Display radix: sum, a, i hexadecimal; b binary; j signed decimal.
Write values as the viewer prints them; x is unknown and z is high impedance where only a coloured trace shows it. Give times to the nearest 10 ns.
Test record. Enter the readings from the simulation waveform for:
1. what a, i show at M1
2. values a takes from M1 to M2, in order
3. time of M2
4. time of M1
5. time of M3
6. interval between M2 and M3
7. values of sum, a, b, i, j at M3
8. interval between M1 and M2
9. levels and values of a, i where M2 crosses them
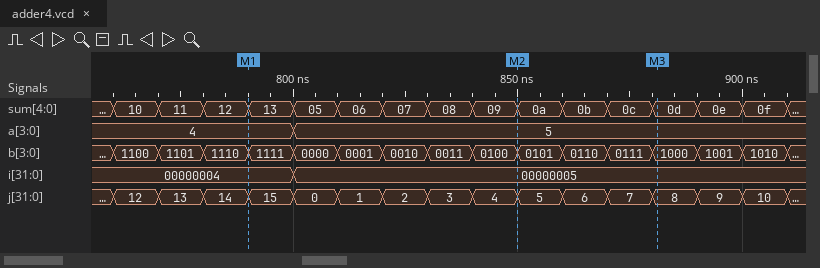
a=4, i=00000004
4, 5
850 ns
790 ns
880 ns
30 ns
sum=0d, a=5, b=1000, i=00000005, j=8
60 ns
a=5, i=00000005
